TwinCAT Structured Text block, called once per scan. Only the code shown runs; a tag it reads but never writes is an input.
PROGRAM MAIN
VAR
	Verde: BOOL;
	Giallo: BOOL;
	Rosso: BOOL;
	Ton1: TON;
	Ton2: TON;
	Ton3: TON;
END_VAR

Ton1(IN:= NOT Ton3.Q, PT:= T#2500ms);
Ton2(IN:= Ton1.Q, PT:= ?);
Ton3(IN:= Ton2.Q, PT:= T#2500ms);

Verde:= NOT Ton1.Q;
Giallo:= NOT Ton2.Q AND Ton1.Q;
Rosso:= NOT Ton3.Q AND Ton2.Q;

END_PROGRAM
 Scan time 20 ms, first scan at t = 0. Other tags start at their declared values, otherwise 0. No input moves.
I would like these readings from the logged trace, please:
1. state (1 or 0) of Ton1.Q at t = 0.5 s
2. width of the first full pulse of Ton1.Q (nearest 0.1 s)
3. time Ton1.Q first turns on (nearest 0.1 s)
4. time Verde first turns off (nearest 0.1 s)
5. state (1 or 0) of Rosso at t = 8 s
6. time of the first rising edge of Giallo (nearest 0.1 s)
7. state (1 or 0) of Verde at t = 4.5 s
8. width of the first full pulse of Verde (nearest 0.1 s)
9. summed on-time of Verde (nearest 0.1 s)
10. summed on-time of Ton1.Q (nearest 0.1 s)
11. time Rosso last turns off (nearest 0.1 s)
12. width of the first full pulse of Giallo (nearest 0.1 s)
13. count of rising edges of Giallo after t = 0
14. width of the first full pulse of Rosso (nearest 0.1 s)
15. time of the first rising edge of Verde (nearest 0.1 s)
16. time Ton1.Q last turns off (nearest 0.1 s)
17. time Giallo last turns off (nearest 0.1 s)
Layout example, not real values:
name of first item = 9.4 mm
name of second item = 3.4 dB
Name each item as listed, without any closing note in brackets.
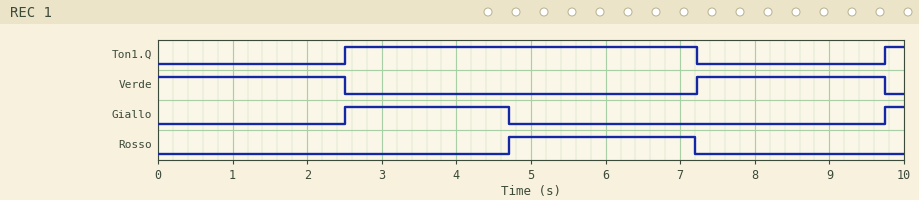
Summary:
state (1 or 0) of Ton1.Q at t = 0.5 s = 0
width of the first full pulse of Ton1.Q = 4.7 s
time Ton1.Q first turns on = 2.5 s
time Verde first turns off = 2.5 s
state (1 or 0) of Rosso at t = 8 s = 0
time of the first rising edge of Giallo = 2.5 s
state (1 or 0) of Verde at t = 4.5 s = 0
width of the first full pulse of Verde = 2.5 s
summed on-time of Verde = 5.0 s
summed on-time of Ton1.Q = 5.0 s
time Rosso last turns off = 7.2 s
width of the first full pulse of Giallo = 2.2 s
count of rising edges of Giallo after t = 0 = 2
width of the first full pulse of Rosso = 2.5 s
time of the first rising edge of Verde = 7.2 s
time Ton1.Q last turns off = 7.2 s
time Giallo last turns off = 4.7 s
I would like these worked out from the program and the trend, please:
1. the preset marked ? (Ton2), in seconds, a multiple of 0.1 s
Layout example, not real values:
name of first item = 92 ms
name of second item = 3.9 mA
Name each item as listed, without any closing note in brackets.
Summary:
the preset marked ? (Ton2), in seconds, a multiple of 0.1 s = 2.2 s
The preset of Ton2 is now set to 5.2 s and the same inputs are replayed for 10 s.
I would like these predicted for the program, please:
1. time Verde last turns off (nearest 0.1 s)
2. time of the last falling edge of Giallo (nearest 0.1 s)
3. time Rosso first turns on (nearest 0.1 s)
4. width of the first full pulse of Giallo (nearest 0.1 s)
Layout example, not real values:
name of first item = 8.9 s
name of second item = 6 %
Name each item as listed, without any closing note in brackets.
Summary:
time Verde last turns off = 2.5 s
time of the last falling edge of Giallo = 7.7 s
time Rosso first turns on = 7.7 s
width of the first full pulse of Giallo = 5.2 s
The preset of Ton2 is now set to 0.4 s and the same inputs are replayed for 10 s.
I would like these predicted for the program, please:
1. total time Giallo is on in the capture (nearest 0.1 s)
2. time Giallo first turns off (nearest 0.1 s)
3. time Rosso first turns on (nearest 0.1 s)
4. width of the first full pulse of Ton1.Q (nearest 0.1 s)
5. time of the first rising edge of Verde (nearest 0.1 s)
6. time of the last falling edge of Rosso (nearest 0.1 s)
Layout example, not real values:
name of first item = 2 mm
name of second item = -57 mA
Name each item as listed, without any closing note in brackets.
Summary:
total time Giallo is on in the capture = 0.8 s
time Giallo first turns off = 2.9 s
time Rosso first turns on = 2.9 s
width of the first full pulse of Ton1.Q = 2.9 s
time of the first rising edge of Verde = 5.4 s
time of the last falling edge of Rosso = 5.4 s
